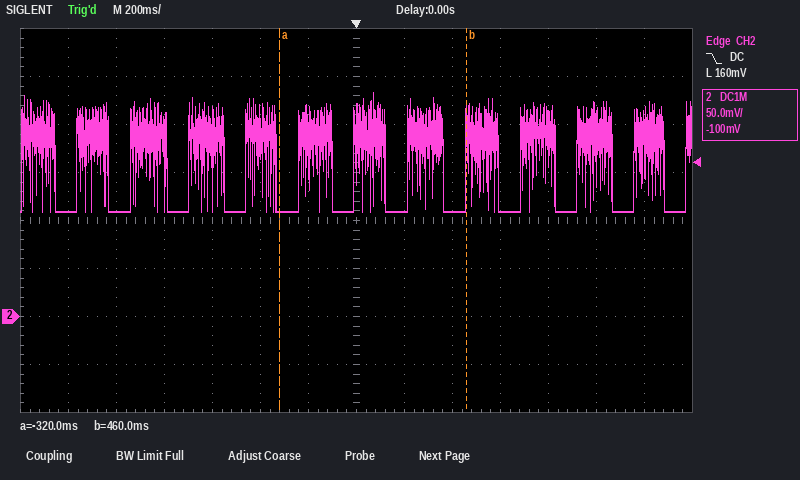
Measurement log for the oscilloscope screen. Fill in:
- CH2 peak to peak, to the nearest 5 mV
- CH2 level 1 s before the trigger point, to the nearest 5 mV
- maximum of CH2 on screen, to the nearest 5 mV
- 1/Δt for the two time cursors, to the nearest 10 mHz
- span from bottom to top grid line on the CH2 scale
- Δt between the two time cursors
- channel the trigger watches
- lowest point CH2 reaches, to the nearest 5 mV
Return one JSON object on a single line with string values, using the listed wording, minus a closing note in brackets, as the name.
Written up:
{"CH2 peak to peak, to the nearest 5 mV": "125 mV", "CH2 level 1 s before the trigger point, to the nearest 5 mV": "110 mV", "maximum of CH2 on screen, to the nearest 5 mV": "235 mV", "1/Δt for the two time cursors, to the nearest 10 mHz": "1.28 Hz", "span from bottom to top grid line on the CH2 scale": "400 mV", "Δt between the two time cursors": "780 ms", "channel the trigger watches": "CH2", "lowest point CH2 reaches, to the nearest 5 mV": "110 mV"}
